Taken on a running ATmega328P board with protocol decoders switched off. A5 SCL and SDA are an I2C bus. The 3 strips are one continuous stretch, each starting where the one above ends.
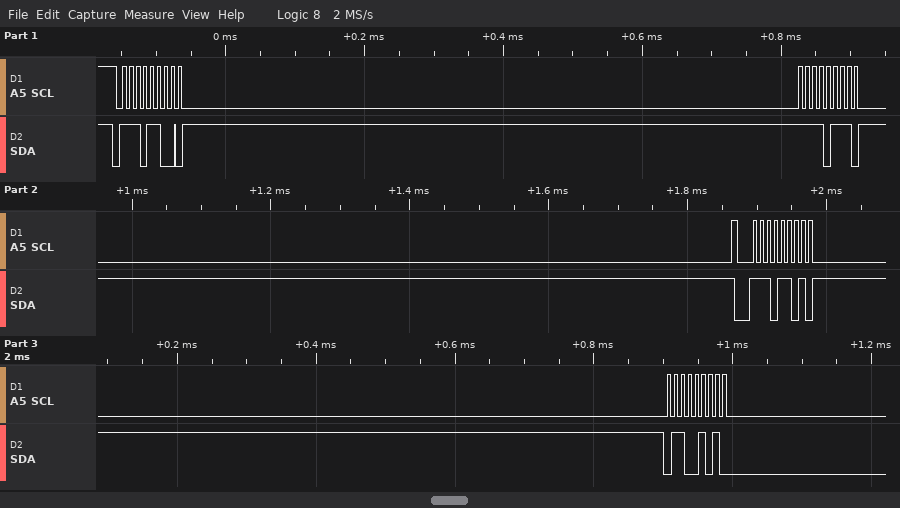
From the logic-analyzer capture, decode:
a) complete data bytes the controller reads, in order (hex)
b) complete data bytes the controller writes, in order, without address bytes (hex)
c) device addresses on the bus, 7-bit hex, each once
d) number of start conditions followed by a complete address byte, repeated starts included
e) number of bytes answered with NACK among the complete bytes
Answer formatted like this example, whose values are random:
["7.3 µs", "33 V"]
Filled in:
["65", "F7", "0x76", "2", "0"]
